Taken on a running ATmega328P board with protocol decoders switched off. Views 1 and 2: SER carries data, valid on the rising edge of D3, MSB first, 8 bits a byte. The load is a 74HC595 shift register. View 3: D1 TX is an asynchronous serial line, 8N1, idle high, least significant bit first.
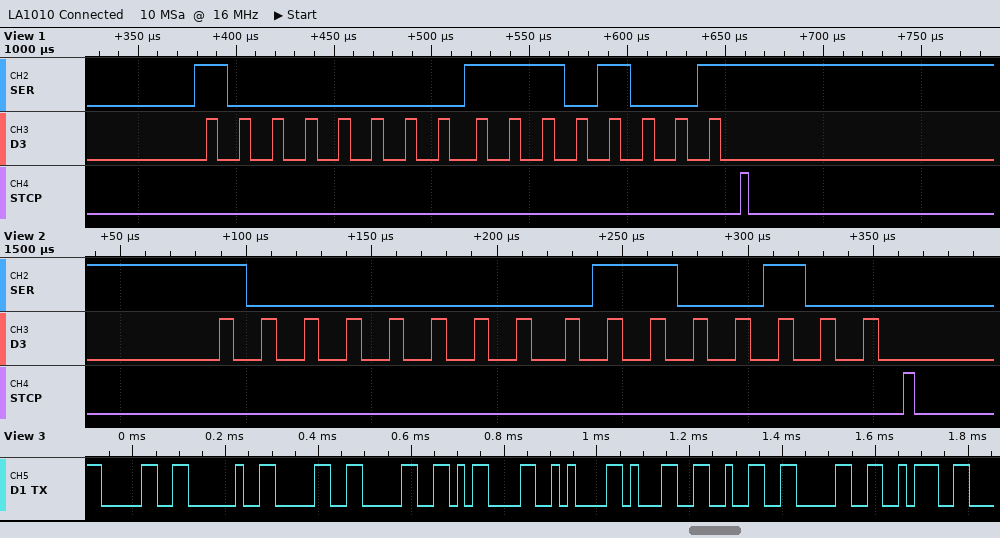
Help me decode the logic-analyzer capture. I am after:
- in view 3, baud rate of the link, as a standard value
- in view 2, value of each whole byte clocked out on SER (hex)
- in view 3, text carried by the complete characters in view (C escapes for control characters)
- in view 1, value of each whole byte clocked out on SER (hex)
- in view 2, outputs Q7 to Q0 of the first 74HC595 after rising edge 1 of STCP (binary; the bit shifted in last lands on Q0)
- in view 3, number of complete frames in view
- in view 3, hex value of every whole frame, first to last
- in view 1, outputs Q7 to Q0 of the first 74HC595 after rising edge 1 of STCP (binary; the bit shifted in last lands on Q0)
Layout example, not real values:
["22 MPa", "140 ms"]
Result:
["57600 baud", "80 64", "\"0 00\\r\\n120:\"", "80 E9", "01100100", "10", "30 20 30 30 0D 0A 31 32 30 3A", "11101001"]
